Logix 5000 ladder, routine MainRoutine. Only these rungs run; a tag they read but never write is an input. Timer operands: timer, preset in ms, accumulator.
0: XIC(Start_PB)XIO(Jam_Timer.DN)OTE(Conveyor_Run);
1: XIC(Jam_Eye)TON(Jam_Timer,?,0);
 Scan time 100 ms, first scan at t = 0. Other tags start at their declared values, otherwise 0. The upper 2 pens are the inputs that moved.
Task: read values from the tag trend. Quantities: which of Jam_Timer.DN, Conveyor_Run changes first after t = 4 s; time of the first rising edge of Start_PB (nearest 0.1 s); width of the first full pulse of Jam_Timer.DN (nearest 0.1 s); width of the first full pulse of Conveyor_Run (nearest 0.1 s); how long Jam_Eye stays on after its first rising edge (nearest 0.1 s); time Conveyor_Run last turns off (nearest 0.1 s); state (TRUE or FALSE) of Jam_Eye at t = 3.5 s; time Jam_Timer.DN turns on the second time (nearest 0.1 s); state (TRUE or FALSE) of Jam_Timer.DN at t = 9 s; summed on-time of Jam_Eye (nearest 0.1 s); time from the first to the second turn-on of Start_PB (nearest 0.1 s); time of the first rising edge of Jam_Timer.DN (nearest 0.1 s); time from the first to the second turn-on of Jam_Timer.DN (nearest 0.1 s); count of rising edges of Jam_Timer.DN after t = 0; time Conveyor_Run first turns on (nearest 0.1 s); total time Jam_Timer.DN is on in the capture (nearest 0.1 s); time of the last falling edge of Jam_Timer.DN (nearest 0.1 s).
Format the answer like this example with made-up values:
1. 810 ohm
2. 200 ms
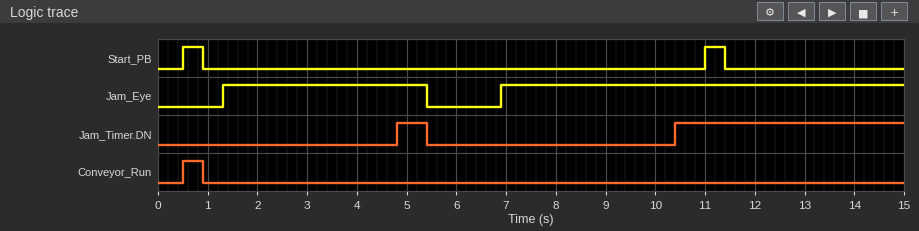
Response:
1. Jam_Timer.DN
2. 0.5 s
3. 0.6 s
4. 0.4 s
5. 4.1 s
6. 0.9 s
7. TRUE
8. 10.4 s
9. FALSE
10. 12.2 s
11. 10.5 s
12. 4.8 s
13. 5.6 s
14. 2
15. 0.5 s
16. 5.2 s
17. 5.4 s
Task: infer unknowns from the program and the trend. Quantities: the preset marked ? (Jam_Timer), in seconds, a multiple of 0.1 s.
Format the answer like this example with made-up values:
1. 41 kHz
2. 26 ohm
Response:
1. 3.5 s
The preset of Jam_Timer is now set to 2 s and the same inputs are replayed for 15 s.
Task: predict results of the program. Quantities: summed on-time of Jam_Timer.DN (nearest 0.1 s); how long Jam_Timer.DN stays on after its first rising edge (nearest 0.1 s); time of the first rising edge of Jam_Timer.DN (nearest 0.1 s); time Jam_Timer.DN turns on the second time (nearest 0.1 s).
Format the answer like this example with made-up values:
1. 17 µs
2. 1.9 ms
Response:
1. 8.2 s
2. 2.1 s
3. 3.3 s
4. 8.9 s
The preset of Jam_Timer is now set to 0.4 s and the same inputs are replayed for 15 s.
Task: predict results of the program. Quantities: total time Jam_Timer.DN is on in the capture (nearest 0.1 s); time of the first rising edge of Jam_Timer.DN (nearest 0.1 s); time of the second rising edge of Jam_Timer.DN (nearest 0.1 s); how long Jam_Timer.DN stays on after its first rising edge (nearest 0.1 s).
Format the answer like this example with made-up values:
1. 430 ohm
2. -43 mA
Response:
1. 11.4 s
2. 1.7 s
3. 7.3 s
4. 3.7 s
